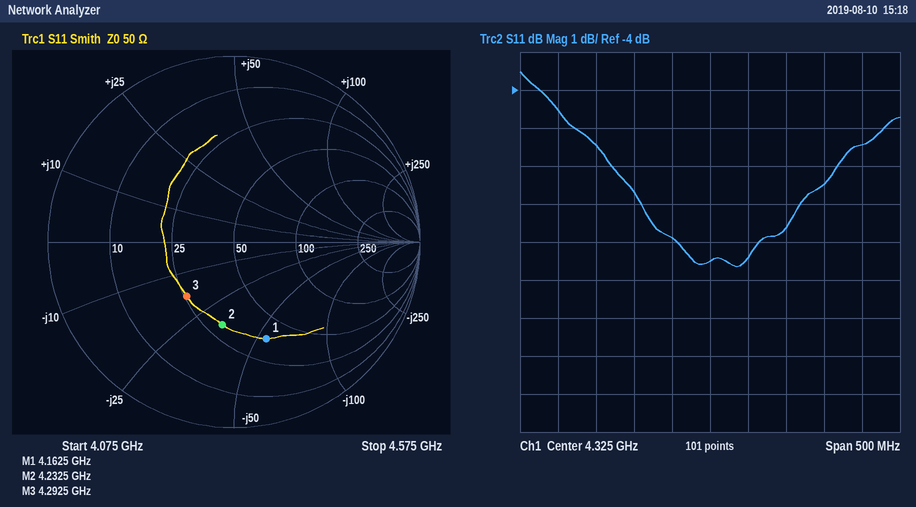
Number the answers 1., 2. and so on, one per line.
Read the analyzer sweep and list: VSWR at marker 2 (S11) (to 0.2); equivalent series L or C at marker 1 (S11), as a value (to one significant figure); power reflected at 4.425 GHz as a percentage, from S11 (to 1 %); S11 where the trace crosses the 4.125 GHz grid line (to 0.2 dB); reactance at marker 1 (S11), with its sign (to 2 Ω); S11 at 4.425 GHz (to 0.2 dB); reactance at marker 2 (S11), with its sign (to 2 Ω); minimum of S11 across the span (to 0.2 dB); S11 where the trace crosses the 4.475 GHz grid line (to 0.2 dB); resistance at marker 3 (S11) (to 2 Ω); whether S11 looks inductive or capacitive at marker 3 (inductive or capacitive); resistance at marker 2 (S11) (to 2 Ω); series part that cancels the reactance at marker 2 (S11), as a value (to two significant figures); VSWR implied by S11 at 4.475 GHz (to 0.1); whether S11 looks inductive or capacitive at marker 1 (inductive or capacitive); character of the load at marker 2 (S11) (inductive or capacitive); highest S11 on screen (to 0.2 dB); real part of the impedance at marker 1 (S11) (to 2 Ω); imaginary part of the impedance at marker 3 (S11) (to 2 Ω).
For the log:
1. 2.6
2. 700 fF
3. 17 %
4. -4.6 dB
5. -54 Ω
6. -7.6 dB
7. -34 Ω
8. -8.6 dB
9. -6.4 dB
10. 26 Ω
11. capacitive
12. 30 Ω
13. 1.3 nH
14. 2.8
15. capacitive
16. capacitive
17. -3.6 dB
18. 36 Ω
19. -18 Ω
